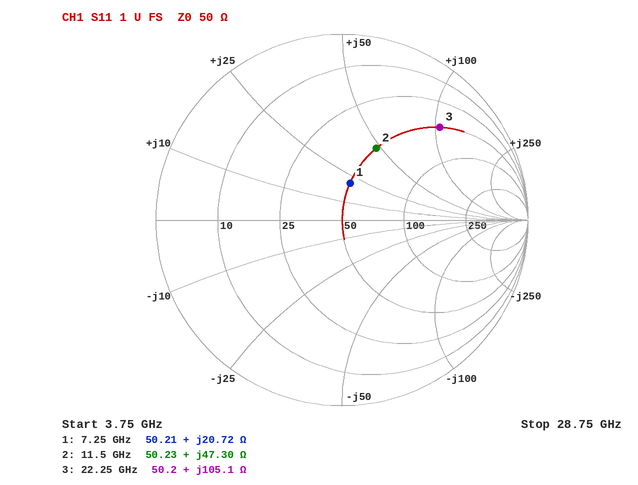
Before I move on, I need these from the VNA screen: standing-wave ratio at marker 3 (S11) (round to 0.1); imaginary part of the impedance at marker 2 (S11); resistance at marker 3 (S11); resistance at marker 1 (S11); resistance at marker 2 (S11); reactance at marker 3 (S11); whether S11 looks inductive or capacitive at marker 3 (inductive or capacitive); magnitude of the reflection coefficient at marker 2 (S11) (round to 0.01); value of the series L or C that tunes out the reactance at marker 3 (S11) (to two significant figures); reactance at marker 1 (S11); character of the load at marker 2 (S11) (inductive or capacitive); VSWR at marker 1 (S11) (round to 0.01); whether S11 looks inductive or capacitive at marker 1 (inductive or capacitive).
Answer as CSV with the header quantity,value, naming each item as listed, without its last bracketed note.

quantity,value
standing-wave ratio at marker 3 (S11),6.2
imaginary part of the impedance at marker 2,+47.30 Ω
resistance at marker 3,50.2 Ω
resistance at marker 1,50.21 Ω
resistance at marker 2,50.23 Ω
reactance at marker 3,+105.1 Ω
whether S11 looks inductive or capacitive at marker 3,inductive
magnitude of the reflection coefficient at marker 2 (S11),0.43
value of the series L or C that tunes out the reactance at marker 3 (S11),68 fF
reactance at marker 1,+20.72 Ω
character of the load at marker 2 (S11),inductive
VSWR at marker 1 (S11),1.51
whether S11 looks inductive or capacitive at marker 1,inductive
